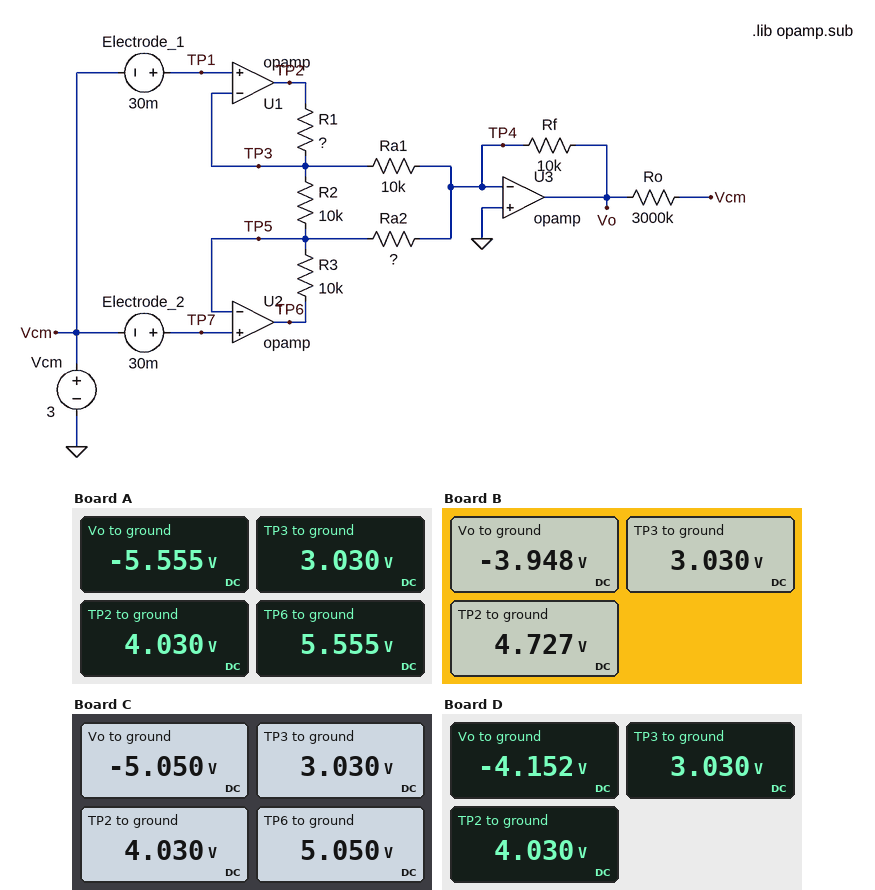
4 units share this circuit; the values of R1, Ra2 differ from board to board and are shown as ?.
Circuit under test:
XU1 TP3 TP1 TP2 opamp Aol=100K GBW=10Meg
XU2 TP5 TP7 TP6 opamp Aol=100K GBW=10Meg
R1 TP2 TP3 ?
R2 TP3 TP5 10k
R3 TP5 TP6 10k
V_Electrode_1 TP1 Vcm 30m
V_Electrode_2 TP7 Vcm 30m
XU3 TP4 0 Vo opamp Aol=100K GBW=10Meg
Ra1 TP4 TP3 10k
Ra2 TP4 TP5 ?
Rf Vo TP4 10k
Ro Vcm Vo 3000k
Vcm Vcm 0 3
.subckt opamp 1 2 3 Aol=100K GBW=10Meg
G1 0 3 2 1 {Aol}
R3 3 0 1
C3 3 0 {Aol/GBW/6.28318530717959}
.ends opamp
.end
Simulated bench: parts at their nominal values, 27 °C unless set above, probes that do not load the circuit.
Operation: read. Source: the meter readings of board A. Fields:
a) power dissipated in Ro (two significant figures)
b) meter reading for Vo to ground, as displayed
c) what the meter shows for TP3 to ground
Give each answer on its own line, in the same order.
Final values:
24 µW
-5.555 V
3.030 V
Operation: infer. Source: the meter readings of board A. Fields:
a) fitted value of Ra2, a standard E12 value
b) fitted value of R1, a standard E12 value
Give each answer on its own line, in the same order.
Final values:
12 kΩ
3.3 kΩ
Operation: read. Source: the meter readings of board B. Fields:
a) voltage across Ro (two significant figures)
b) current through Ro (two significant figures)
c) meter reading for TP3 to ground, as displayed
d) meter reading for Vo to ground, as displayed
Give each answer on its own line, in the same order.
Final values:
6.9 V
2.3 µA
3.030 V
-3.948 V
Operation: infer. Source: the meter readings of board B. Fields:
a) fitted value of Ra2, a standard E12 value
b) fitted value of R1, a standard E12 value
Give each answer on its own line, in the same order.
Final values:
33 kΩ
5.6 kΩ
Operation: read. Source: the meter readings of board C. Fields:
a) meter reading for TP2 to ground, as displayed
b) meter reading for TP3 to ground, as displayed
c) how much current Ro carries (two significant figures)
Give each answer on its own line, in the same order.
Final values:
4.030 V
3.030 V
2.7 µA
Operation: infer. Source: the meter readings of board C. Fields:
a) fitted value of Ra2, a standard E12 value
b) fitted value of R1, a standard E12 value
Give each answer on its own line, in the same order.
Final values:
15 kΩ
3.3 kΩ
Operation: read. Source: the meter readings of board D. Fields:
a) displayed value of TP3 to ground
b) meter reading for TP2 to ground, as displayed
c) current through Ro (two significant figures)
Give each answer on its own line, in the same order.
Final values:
3.030 V
4.030 V
2.4 µA
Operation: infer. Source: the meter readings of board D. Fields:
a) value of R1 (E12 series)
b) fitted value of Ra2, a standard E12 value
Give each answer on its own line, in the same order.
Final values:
3.3 kΩ
27 kΩ
